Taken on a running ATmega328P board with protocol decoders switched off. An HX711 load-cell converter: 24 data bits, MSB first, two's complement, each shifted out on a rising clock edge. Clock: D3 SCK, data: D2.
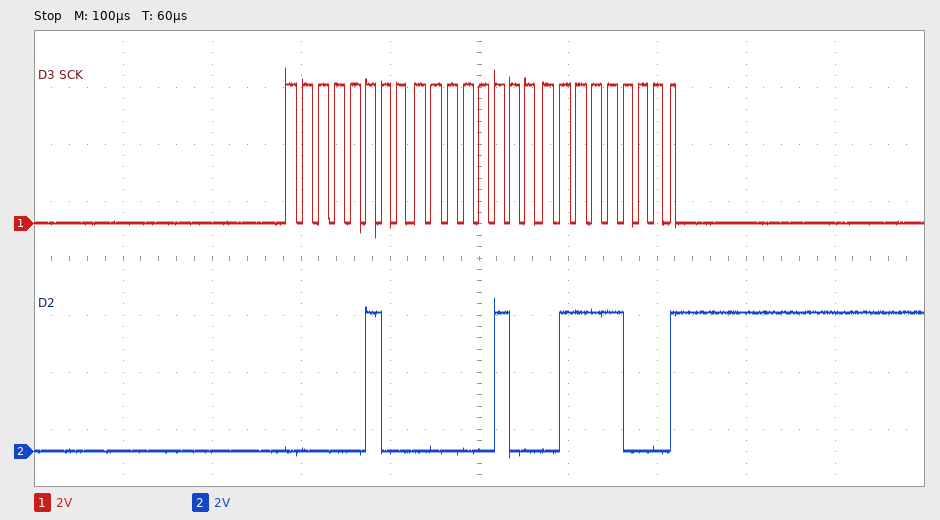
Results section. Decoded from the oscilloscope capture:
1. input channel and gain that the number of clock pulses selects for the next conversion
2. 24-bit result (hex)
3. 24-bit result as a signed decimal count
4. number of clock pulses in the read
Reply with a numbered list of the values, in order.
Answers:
1. channel A, gain 128
2. 0x040478
3. 263288
4. 25
